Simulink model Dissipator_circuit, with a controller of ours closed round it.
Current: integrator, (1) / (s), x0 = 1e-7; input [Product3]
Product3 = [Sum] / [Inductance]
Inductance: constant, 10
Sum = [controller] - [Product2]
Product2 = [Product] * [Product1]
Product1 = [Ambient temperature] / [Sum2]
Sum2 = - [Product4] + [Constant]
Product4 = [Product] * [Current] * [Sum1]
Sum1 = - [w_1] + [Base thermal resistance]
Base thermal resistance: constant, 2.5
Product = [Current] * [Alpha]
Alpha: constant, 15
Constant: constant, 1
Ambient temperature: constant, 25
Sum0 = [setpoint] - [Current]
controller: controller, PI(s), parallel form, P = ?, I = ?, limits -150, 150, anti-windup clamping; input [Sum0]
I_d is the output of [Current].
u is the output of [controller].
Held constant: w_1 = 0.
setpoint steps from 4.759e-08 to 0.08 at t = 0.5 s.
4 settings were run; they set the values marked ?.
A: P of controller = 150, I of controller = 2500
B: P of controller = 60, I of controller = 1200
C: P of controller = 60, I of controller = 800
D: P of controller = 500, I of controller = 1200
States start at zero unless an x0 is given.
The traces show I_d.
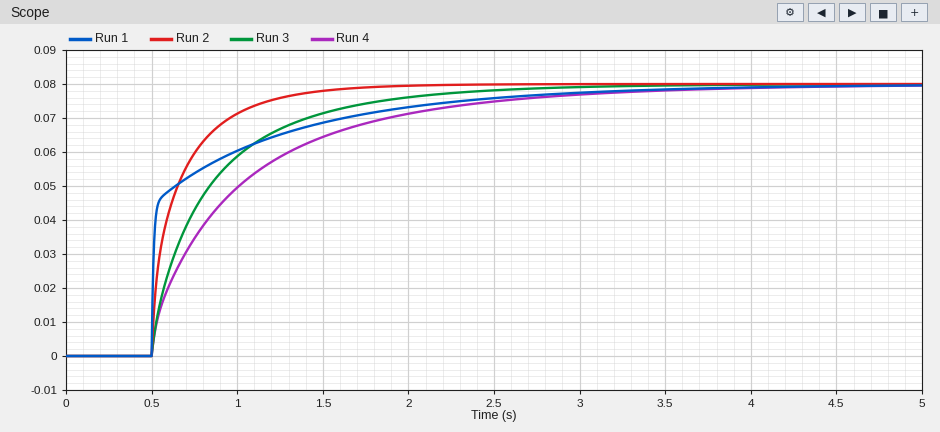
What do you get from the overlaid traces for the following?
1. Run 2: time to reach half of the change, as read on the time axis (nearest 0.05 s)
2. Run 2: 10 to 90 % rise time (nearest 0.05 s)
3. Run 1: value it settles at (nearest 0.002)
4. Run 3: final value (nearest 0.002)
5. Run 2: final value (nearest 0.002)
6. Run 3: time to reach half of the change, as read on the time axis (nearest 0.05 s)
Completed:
0.60 s
0.50 s
0.080
0.080
0.080
0.70 s
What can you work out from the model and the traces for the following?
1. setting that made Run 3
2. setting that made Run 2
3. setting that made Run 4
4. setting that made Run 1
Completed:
B
A
C
D
